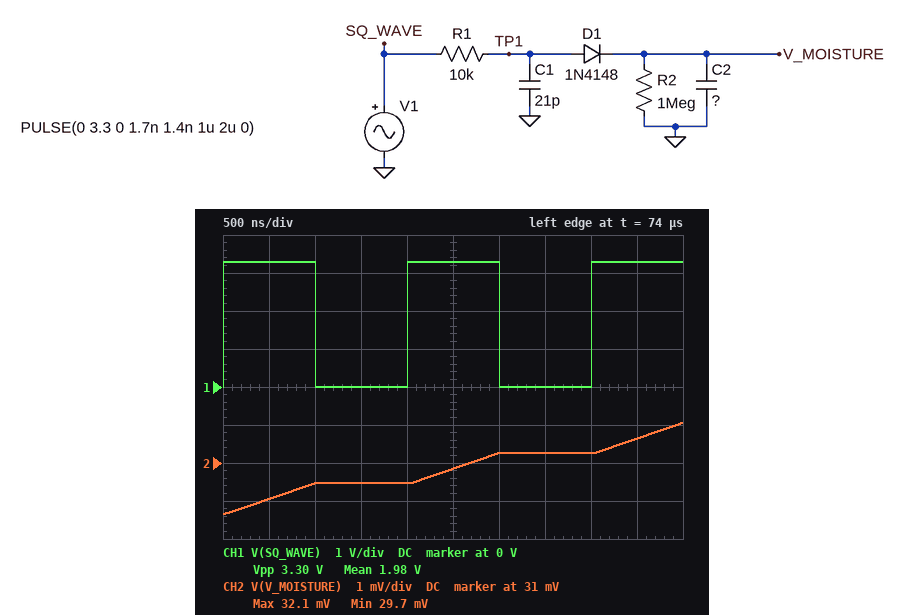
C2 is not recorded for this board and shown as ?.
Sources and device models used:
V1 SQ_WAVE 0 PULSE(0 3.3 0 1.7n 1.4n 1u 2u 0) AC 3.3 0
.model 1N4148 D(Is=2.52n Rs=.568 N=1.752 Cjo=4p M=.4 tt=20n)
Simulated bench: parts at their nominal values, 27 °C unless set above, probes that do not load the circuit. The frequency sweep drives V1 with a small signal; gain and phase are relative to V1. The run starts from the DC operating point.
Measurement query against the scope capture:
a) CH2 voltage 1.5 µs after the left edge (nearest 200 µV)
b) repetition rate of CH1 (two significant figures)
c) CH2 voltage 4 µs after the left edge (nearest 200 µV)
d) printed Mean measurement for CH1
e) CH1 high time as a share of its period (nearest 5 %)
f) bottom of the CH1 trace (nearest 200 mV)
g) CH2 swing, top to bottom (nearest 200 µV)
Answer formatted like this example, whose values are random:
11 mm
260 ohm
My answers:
30.4 mV
500 kHz
31.2 mV
1.98 V
50 %
0 V
2.4 mV
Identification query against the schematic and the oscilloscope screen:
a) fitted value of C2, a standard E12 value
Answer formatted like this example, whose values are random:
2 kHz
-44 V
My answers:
330 nF
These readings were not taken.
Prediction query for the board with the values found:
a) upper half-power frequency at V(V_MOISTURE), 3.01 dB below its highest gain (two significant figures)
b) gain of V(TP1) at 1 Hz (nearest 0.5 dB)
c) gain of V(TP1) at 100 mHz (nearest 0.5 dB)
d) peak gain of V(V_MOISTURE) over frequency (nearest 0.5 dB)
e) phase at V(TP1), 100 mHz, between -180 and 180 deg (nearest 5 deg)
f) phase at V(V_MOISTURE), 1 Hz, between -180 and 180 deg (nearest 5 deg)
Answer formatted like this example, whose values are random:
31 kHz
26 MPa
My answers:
510 mHz
0 dB
0 dB
-25.5 dB
0 deg
-65 deg
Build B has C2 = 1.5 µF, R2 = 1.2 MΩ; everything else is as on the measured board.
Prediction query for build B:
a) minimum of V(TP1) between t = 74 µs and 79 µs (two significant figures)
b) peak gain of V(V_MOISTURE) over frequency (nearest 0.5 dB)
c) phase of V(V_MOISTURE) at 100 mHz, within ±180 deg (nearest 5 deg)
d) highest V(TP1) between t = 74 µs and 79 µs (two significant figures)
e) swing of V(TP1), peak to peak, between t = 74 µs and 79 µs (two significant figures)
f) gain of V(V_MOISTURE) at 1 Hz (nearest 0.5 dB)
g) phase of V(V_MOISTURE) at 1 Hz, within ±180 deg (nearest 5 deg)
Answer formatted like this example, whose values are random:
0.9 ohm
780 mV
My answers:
9.7 mV
-24.0 dB
-45 deg
530 mV
520 mV
-44.5 dB
-85 deg
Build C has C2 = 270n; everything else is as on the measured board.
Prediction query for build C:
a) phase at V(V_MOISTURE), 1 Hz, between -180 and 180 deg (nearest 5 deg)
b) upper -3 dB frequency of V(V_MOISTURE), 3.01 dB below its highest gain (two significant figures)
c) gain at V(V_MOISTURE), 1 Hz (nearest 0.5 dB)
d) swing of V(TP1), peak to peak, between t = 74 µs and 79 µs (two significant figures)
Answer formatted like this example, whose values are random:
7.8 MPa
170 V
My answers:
-60 deg
620 mHz
-31.0 dB
550 mV
